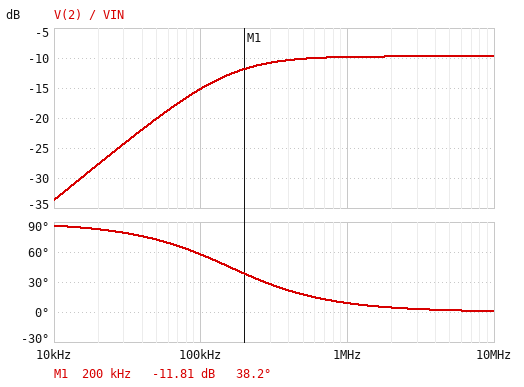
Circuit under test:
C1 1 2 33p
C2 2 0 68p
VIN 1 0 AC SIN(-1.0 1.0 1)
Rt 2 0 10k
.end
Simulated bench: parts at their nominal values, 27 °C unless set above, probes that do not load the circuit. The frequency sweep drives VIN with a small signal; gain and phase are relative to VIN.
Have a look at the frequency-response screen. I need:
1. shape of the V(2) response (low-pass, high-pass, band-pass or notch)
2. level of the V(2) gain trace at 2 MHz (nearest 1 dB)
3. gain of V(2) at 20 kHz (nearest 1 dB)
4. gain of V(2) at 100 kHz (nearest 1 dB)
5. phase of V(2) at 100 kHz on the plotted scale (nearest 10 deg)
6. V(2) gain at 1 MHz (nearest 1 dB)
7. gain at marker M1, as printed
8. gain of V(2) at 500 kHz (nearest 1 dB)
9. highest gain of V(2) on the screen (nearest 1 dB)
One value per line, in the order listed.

high-pass
-10 dB
-28 dB
-15 dB
60 deg
-10 dB
-11.81 dB
-10 dB
-10 dB
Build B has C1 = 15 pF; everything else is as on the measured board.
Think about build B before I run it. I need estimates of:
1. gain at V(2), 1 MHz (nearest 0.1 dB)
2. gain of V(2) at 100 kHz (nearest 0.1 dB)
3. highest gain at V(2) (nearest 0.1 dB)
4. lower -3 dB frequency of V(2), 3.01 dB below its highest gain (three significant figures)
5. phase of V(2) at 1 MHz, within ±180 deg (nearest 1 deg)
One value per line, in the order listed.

-15.0 dB
-21.6 dB
-14.9 dB
192 kHz
11 deg
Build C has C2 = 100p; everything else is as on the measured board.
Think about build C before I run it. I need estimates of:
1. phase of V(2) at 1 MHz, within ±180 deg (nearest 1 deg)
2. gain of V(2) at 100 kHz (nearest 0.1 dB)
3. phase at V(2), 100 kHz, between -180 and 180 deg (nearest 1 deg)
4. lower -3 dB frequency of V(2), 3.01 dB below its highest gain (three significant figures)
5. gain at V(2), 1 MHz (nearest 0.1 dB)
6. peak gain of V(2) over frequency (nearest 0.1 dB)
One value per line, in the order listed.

7 deg
-16.0 dB
50 deg
120 kHz
-12.2 dB
-12.1 dB
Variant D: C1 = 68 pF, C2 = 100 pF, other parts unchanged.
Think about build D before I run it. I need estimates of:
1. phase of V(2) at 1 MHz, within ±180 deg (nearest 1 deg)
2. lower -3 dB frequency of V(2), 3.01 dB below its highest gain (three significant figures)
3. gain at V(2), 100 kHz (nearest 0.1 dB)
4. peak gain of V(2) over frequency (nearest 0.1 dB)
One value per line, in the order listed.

5 deg
94.7 kHz
-10.6 dB
-7.9 dB
